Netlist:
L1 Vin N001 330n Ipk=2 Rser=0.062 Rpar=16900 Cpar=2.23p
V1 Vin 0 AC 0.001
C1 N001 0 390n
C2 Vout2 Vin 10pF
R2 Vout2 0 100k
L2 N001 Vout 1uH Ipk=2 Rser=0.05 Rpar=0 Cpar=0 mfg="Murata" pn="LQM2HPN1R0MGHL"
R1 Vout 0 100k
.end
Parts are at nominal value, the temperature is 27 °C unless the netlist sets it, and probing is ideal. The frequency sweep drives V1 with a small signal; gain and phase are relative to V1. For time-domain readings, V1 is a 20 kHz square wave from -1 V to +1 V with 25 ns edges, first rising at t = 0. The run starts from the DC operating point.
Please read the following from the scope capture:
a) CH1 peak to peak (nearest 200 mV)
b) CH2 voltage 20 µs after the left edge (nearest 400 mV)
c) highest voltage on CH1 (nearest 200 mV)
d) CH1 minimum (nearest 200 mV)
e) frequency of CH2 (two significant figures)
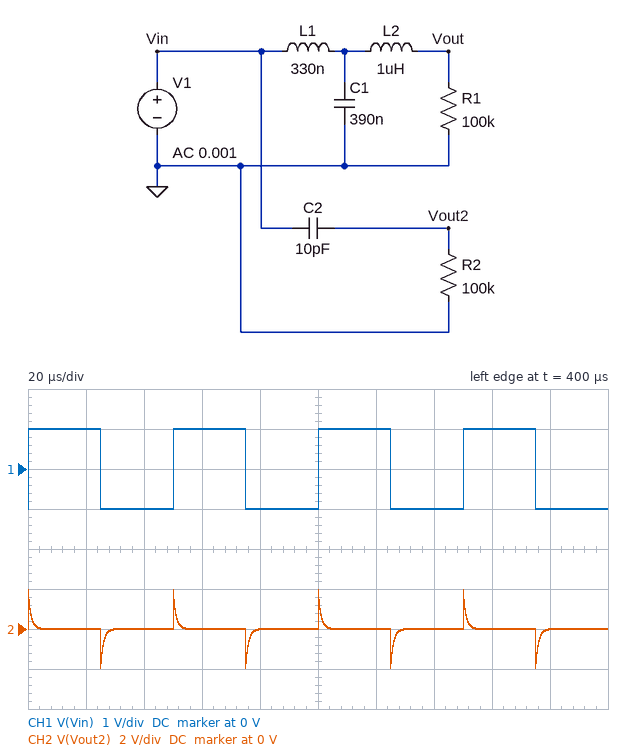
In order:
2.0 V
0 V
1.0 V
-1.0 V
20 kHz
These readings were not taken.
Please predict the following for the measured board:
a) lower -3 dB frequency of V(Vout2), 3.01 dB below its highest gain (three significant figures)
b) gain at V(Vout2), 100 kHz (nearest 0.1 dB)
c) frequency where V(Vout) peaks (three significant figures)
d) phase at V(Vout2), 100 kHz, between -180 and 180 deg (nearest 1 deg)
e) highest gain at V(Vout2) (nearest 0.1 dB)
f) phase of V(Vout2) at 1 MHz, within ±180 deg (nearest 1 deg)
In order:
159 kHz
-5.5 dB
443 kHz
58 deg
0 dB
9 deg
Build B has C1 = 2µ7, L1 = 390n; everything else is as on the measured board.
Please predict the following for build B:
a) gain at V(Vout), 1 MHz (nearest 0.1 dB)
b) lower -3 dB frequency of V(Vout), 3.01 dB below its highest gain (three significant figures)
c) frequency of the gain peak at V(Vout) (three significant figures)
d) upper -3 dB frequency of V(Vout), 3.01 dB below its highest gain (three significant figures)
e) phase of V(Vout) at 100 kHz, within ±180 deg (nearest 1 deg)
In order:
-32.2 dB
141 kHz
154 kHz
166 kHz
-10 deg
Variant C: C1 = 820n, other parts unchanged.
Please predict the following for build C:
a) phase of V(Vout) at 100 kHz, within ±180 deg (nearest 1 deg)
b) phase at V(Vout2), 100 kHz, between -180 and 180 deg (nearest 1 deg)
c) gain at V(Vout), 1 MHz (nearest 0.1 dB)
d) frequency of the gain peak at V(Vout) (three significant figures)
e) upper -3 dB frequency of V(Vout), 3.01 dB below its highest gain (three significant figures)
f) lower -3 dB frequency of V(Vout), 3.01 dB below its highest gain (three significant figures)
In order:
-2 deg
58 deg
-19.7 dB
305 kHz
320 kHz
290 kHz
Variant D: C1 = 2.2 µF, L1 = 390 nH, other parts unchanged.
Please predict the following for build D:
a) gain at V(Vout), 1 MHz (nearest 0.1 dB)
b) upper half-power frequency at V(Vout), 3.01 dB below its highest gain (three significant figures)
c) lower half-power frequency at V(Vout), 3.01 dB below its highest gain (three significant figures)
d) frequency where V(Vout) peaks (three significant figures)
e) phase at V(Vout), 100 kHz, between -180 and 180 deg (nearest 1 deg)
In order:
-30.3 dB
183 kHz
158 kHz
171 kHz
-7 deg
